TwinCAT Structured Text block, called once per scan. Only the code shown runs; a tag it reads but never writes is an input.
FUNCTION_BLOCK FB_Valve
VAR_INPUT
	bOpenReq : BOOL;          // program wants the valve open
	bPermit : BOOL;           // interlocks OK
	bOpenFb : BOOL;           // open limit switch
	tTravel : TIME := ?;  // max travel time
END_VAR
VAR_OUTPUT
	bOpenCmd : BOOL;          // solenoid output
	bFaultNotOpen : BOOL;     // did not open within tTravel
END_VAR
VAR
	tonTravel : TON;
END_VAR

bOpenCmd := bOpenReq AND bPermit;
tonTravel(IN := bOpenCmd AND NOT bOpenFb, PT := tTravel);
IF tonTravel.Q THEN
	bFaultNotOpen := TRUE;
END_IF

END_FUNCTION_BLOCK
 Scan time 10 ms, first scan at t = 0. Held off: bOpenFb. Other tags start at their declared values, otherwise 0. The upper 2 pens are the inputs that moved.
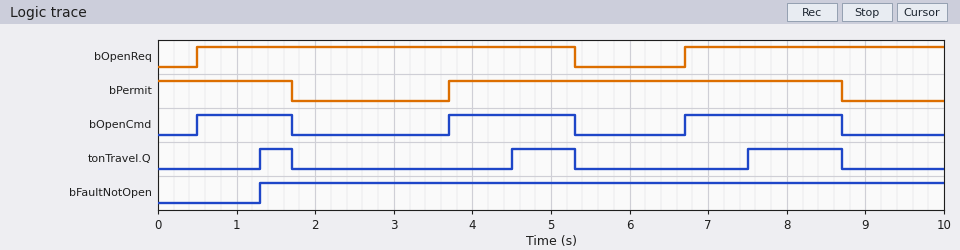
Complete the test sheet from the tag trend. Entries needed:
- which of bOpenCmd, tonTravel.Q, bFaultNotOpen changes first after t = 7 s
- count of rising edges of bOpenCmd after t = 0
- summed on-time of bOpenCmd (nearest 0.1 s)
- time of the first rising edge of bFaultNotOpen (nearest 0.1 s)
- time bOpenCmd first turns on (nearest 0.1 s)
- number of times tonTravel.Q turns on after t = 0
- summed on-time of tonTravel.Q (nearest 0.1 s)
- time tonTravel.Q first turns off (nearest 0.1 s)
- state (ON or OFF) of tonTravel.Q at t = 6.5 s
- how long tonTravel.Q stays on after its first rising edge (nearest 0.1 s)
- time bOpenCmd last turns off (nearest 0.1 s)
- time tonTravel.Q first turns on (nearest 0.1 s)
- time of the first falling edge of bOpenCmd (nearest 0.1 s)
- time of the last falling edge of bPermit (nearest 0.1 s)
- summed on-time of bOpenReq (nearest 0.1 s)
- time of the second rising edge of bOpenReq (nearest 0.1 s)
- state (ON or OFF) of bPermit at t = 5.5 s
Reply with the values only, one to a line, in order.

tonTravel.Q
3
4.8 s
1.3 s
0.5 s
3
2.4 s
1.7 s
OFF
0.4 s
8.7 s
1.3 s
1.7 s
8.7 s
8.1 s
6.7 s
ON
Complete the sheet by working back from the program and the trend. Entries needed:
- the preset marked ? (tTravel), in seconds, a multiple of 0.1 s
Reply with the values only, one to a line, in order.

0.8 s
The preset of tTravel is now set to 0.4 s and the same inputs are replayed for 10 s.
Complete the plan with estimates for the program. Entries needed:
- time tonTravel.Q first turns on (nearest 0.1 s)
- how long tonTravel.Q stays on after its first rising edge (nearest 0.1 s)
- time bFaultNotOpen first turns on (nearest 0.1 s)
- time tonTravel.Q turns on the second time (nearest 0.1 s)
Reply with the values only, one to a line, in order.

0.9 s
0.8 s
0.9 s
4.1 s
